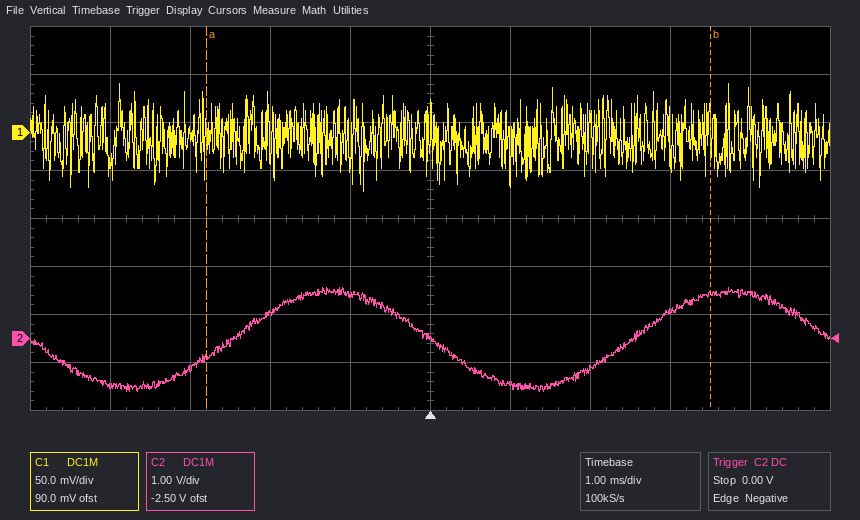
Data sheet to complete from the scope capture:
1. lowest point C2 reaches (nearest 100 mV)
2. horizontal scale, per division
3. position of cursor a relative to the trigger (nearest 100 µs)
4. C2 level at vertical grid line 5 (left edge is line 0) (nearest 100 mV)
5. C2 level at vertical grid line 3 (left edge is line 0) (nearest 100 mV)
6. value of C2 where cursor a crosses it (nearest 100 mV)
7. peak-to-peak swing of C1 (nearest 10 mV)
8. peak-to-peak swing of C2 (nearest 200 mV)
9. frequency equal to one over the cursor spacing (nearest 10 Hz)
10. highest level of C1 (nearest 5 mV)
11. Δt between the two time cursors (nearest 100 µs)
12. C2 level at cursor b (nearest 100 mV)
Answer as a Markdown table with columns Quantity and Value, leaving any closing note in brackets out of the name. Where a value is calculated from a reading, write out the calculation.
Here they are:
| Quantity | Value |
|---|---|
| lowest point C2 reaches | -1.1 V |
| horizontal scale, per division | 1 ms |
| position of cursor a relative to the trigger | -2.8 ms |
| C2 level at vertical grid line 5 (left edge is line 0) | 0.0 V |
| C2 level at vertical grid line 3 (left edge is line 0) | 500 mV |
| value of C2 where cursor a crosses it | -400 mV |
| peak-to-peak swing of C1 | 110 mV |
| peak-to-peak swing of C2 | 2.2 V |
| frequency equal to one over the cursor spacing | 1 / 6.3 ms ≈ 160 Hz |
| highest level of C1 | 50 mV |
| Δt between the two time cursors | 6.3 ms |
| C2 level at cursor b | 900 mV |
